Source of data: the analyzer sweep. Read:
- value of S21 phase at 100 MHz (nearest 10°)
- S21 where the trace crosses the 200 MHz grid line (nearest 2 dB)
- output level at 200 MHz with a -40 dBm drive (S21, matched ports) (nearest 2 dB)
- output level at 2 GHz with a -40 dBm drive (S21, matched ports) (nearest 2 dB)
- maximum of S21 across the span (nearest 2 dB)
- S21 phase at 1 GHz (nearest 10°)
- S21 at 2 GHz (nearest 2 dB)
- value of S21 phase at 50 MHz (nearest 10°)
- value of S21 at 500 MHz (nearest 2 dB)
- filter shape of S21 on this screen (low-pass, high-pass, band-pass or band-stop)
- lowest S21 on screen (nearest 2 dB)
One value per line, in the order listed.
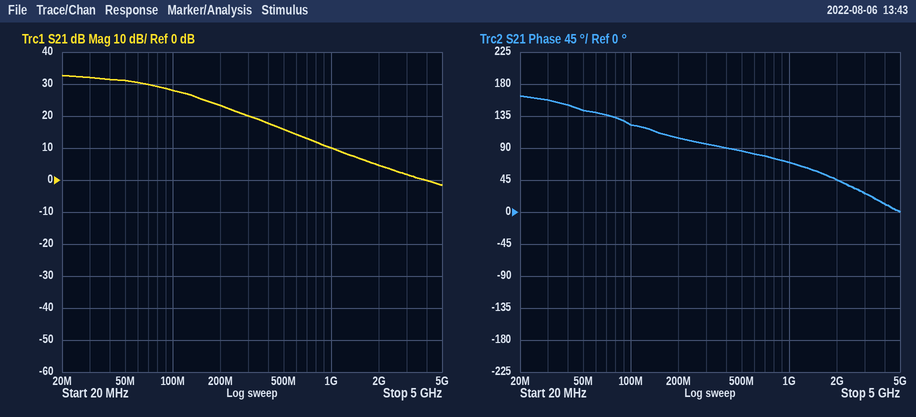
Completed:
120°
24 dB
-16 dBm
-36 dBm
32 dB
70°
4 dB
140°
16 dB
low-pass
-2 dB
